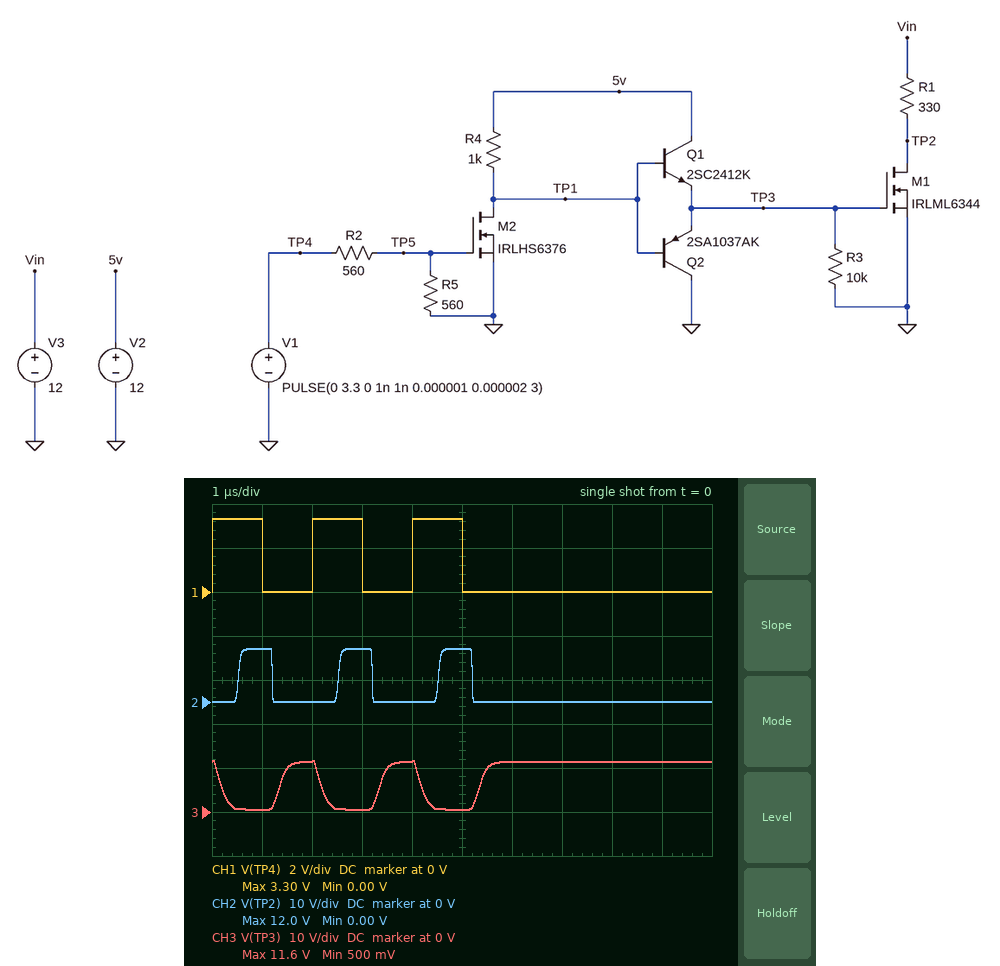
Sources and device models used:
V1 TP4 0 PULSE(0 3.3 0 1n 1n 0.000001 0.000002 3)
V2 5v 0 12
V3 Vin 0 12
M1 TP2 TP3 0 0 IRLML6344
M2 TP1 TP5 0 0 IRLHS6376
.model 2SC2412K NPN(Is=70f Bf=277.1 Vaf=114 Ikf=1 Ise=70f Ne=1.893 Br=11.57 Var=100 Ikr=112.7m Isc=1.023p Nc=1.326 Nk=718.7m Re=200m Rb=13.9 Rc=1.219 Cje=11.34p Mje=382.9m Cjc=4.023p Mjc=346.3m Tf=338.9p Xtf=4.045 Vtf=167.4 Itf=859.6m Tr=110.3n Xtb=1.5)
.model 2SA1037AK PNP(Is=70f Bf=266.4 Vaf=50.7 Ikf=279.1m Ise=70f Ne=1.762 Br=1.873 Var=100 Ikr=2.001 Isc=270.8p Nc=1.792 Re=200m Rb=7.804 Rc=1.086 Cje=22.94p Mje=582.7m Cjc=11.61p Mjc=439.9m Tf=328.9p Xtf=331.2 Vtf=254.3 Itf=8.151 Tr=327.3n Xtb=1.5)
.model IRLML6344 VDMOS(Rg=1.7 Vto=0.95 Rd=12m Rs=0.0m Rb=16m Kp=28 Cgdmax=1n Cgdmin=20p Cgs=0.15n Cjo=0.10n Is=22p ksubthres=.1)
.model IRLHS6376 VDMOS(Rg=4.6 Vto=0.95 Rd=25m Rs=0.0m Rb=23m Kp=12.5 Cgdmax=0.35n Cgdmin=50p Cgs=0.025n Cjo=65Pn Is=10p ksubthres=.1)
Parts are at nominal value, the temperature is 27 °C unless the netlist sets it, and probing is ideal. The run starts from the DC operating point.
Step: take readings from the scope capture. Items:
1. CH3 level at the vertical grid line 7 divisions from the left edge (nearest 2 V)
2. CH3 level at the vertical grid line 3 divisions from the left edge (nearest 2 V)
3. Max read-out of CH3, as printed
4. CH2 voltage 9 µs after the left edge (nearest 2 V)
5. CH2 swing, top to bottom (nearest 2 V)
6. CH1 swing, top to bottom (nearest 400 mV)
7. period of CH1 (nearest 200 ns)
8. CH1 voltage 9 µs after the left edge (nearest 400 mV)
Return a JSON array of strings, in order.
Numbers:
["12 V", "0 V", "11.6 V", "0 V", "12 V", "3.2 V", "2.0 µs", "0 V"]
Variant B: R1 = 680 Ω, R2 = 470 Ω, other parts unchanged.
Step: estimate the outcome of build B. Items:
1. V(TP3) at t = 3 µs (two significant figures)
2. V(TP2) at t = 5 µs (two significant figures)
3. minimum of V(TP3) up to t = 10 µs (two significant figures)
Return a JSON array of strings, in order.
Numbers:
["490 mV", "12 V", "480 mV"]
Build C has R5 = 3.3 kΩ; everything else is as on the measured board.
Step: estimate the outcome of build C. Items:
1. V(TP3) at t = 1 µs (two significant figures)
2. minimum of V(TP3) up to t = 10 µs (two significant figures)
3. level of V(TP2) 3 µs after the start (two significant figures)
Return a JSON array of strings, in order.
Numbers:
["440 mV", "410 mV", "12 V"]
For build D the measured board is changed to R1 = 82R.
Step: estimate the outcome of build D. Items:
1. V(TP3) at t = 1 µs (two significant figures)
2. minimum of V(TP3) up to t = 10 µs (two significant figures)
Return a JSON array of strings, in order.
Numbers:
["440 mV", "430 mV"]
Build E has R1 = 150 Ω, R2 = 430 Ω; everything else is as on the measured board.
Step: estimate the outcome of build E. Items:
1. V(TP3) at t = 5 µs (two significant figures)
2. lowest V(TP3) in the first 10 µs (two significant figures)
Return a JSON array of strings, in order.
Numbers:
["420 mV", "410 mV"]
